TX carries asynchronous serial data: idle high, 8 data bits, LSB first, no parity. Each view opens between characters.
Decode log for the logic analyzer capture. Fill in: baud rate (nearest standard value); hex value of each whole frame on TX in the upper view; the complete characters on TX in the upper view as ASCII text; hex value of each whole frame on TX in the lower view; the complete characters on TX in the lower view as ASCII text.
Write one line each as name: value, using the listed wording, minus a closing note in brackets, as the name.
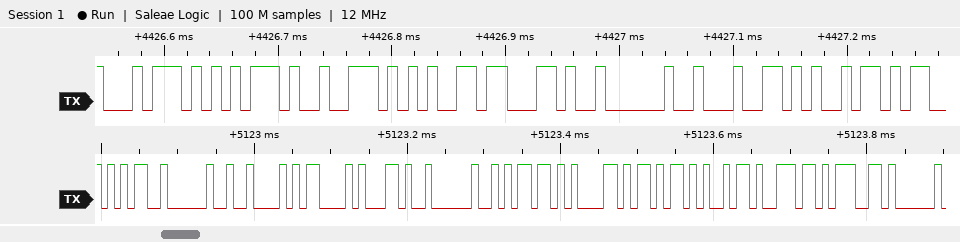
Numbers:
baud rate: 115200 baud
hex value of each whole frame on TX in the upper view: 74, 75, 72, 65, 2C, 20, 64, 69
the complete characters on TX in the upper view as ASCII text: "ture, di"
hex value of each whole frame on TX in the lower view: 35, 20, 42, 43, 2C, 20, 6D, 61, 6B, 69, 6E, 67
the complete characters on TX in the lower view as ASCII text: "5 BC, making"
